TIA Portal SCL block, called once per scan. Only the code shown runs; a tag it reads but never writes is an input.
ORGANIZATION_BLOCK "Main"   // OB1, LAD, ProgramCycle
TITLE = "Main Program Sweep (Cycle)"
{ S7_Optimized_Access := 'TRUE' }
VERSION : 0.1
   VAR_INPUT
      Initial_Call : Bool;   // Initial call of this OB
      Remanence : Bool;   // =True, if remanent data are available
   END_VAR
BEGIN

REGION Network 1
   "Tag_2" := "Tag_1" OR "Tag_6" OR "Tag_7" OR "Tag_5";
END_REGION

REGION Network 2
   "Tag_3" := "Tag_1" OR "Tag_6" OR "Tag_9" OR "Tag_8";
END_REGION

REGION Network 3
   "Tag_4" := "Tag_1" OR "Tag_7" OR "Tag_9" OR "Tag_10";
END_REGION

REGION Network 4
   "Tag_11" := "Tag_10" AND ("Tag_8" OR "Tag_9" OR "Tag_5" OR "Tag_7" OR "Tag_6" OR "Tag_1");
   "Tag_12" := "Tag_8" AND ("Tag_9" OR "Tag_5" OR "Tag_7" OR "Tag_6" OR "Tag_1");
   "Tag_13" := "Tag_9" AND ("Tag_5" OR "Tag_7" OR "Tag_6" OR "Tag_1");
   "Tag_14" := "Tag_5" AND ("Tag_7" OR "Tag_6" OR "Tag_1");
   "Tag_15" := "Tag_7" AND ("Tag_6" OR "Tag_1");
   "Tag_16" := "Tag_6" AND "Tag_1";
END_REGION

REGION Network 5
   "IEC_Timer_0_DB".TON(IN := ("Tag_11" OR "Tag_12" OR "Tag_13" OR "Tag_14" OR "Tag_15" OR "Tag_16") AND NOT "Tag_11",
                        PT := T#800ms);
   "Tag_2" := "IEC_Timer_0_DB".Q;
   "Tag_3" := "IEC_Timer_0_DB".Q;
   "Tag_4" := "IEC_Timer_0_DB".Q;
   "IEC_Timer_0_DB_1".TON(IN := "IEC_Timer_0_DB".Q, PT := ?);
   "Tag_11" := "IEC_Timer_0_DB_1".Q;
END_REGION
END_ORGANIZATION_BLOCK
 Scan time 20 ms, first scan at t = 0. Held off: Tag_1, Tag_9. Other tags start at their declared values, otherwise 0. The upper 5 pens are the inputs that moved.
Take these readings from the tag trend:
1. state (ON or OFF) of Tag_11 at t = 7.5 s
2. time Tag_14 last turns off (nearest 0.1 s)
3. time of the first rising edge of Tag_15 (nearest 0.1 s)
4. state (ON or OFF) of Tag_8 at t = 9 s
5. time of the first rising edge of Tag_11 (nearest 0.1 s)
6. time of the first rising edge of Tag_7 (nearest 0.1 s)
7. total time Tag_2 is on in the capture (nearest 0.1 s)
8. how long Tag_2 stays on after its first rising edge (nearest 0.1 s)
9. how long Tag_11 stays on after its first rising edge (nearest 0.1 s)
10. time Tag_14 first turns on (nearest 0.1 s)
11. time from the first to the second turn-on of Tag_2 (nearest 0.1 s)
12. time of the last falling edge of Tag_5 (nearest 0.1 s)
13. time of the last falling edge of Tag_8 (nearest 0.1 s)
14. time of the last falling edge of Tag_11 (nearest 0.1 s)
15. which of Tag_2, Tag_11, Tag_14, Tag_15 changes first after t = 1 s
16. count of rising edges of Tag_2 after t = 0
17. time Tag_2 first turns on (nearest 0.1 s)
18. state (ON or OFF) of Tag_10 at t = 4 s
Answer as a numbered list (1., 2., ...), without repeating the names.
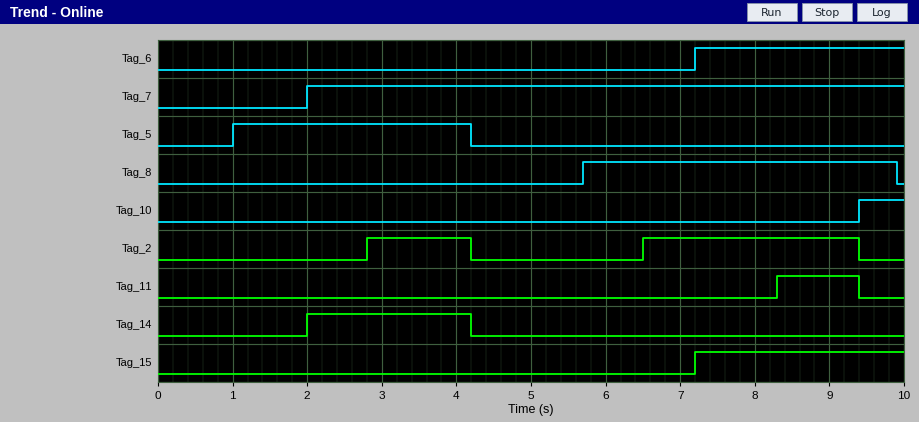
1. OFF
2. 4.2 s
3. 7.2 s
4. ON
5. 8.3 s
6. 2.0 s
7. 4.3 s
8. 1.4 s
9. 1.1 s
10. 2.0 s
11. 3.7 s
12. 4.2 s
13. 9.9 s
14. 9.4 s
15. Tag_14
16. 2
17. 2.8 s
18. OFF
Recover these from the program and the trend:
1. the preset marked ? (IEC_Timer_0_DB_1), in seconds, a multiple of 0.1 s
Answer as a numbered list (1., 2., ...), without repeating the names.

1. 1.8 s
